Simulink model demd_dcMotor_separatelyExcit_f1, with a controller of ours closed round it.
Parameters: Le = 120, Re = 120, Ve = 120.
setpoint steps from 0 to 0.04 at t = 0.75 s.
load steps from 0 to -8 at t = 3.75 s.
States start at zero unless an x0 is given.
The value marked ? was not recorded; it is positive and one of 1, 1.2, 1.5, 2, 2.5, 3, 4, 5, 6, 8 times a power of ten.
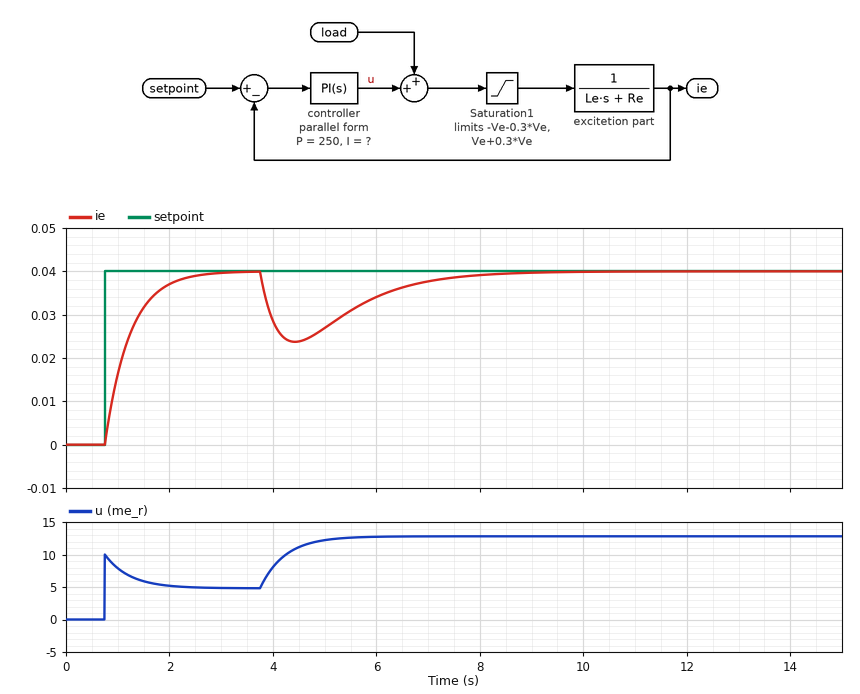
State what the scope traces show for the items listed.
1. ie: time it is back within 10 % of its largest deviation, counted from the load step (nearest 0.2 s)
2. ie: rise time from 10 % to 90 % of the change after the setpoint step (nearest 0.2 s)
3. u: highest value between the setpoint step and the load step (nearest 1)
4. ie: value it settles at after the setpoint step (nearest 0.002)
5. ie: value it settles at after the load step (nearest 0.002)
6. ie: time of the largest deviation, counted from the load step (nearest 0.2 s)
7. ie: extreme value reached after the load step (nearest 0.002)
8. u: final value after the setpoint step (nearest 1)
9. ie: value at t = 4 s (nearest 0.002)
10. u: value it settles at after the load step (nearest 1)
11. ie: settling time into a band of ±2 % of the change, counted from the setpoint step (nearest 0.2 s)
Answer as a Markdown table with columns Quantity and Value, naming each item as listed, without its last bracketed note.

| Quantity | Value |
|---|---|
| ie: time it is back within 10 % of its largest deviation, counted from the load step | 3.6 s |
| ie: rise time from 10 % to 90 % of the change after the setpoint step | 1.0 s |
| u: highest value between the setpoint step and the load step | 10 |
| ie: value it settles at after the setpoint step | 0.040 |
| ie: value it settles at after the load step | 0.040 |
| ie: time of the largest deviation, counted from the load step | 0.6 s |
| ie: extreme value reached after the load step | 0.024 |
| u: final value after the setpoint step | 5 |
| ie: value at t = 4 s | 0.028 |
| u: value it settles at after the load step | 13 |
| ie: settling time into a band of ±2 % of the change, counted from the setpoint step | 1.8 s |
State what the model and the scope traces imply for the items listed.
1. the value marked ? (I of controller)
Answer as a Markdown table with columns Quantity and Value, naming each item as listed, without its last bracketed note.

| Quantity | Value |
|---|---|
| the value marked ? | 250 |
